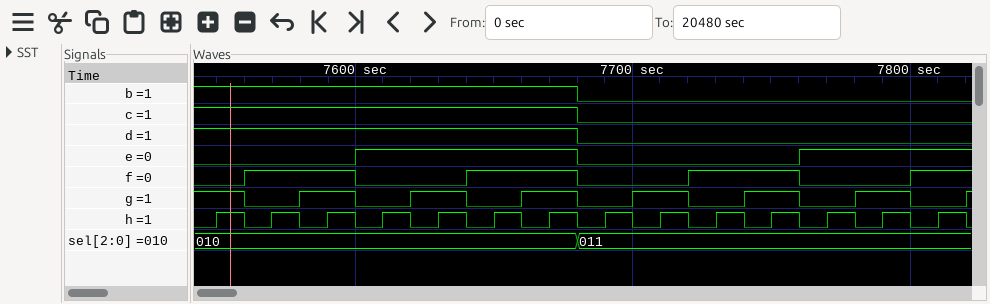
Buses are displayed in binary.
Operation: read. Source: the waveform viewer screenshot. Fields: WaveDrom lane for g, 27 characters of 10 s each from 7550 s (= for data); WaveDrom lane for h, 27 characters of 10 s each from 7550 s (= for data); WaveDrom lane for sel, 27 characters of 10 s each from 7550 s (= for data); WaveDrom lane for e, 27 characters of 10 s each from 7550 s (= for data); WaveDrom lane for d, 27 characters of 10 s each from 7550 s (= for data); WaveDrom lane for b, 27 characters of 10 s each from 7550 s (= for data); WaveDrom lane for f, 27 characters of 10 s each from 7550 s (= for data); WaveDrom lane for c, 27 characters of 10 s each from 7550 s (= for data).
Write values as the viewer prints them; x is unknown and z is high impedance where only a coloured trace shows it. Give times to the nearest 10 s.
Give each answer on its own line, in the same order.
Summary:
{name: 'g', wave: '10.1.0.1.0.1.0.1.0.1.0.1.0.'}
{name: 'h', wave: '101010101010101010101010101'}
{name: 'sel', wave: '=............=.............', data: '010 011'}
{name: 'e', wave: '0....1.......0.......1.....'}
{name: 'd', wave: '1............0.............'}
{name: 'b', wave: '1............0.............'}
{name: 'f', wave: '01...0...1...0...1...0...1.'}
{name: 'c', wave: '1............0.............'}
